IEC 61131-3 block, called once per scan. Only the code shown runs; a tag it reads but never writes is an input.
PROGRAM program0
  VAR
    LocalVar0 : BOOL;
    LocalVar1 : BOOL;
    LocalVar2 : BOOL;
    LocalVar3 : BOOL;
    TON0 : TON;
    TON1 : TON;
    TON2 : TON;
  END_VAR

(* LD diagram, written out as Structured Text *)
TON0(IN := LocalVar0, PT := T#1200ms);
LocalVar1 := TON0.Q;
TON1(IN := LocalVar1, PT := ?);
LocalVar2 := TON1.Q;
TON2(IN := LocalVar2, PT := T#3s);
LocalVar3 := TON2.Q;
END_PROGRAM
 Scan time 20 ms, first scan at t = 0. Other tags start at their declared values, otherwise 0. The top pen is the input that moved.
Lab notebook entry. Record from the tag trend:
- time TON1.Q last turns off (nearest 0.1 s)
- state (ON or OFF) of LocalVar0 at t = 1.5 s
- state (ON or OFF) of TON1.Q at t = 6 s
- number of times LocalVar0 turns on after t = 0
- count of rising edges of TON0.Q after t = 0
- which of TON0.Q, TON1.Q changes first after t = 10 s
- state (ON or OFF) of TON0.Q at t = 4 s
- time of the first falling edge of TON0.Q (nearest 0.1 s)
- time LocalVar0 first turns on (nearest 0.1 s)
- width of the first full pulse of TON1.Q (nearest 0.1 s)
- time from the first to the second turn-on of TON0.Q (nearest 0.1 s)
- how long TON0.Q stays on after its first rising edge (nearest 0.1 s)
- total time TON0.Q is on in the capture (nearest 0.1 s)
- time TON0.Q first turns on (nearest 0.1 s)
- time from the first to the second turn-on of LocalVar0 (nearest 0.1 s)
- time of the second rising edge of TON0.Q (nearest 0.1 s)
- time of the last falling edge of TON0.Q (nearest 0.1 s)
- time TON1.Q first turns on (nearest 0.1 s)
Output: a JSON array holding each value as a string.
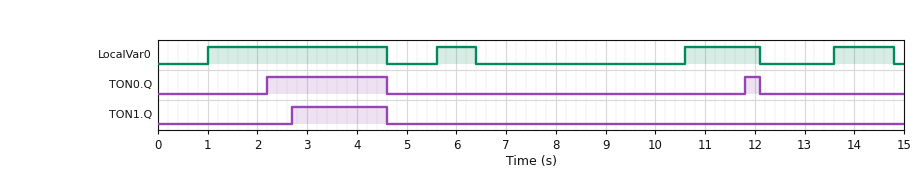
["4.6 s", "ON", "OFF", "4", "2", "TON0.Q", "ON", "4.6 s", "1.0 s", "1.9 s", "9.6 s", "2.4 s", "2.7 s", "2.2 s", "4.6 s", "11.8 s", "12.1 s", "2.7 s"]
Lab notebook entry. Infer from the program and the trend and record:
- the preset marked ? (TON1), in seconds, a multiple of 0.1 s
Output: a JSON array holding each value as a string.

["0.5 s"]
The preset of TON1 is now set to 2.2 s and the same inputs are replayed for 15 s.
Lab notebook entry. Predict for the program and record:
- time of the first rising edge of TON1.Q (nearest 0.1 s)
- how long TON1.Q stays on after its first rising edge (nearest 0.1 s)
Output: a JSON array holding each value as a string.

["4.4 s", "0.2 s"]
